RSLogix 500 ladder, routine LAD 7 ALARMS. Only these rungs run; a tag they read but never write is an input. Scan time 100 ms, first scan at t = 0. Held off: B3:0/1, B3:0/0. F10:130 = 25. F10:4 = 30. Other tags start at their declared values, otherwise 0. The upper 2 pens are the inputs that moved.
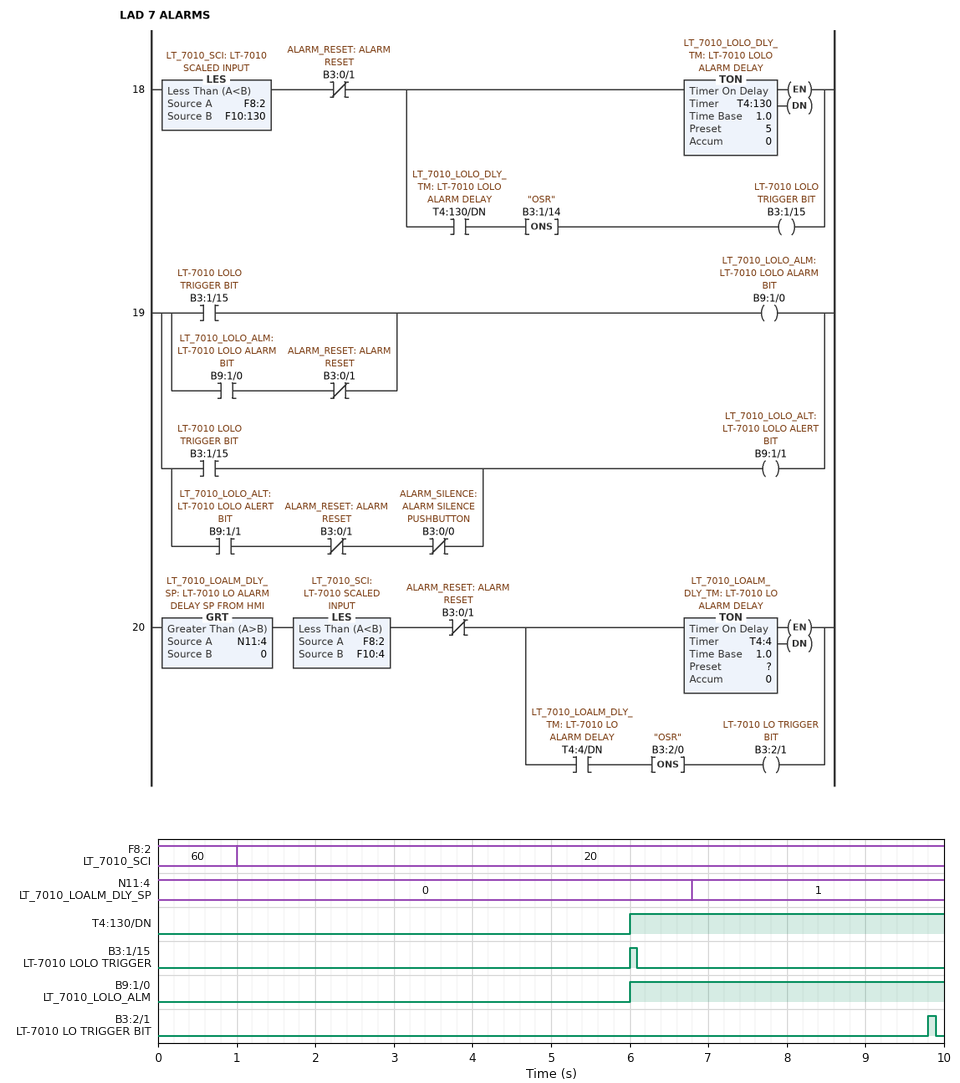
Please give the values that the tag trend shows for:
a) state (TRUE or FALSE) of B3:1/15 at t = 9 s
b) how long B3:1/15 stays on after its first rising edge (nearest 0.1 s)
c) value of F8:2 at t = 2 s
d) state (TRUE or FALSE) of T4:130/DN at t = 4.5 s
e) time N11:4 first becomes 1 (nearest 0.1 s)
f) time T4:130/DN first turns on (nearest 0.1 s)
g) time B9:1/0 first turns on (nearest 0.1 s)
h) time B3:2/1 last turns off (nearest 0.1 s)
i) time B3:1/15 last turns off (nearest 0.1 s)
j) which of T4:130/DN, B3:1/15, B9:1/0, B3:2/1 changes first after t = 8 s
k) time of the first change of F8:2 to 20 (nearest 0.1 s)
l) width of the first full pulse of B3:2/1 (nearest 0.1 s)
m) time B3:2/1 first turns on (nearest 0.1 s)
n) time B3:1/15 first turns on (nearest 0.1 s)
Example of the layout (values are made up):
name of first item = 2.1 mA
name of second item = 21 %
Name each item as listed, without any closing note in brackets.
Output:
state (TRUE or FALSE) of B3:1/15 at t = 9 s = FALSE
how long B3:1/15 stays on after its first rising edge = 0.1 s
value of F8:2 at t = 2 s = 20
state (TRUE or FALSE) of T4:130/DN at t = 4.5 s = FALSE
time N11:4 first becomes 1 = 6.8 s
time T4:130/DN first turns on = 6.0 s
time B9:1/0 first turns on = 6.0 s
time B3:2/1 last turns off = 9.9 s
time B3:1/15 last turns off = 6.1 s
which of T4:130/DN, B3:1/15, B9:1/0, B3:2/1 changes first after t = 8 s = B3:2/1
time of the first change of F8:2 to 20 = 1.0 s
width of the first full pulse of B3:2/1 = 0.1 s
time B3:2/1 first turns on = 9.8 s
time B3:1/15 first turns on = 6.0 s
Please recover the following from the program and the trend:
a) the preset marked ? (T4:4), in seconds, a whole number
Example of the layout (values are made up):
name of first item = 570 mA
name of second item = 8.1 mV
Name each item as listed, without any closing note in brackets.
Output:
the preset marked ? (T4:4), in seconds, a whole number = 3 s
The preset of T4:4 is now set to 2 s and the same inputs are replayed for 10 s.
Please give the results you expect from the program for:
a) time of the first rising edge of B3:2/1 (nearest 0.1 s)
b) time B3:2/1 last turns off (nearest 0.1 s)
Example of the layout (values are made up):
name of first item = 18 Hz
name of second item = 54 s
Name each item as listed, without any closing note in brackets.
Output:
time of the first rising edge of B3:2/1 = 8.8 s
time B3:2/1 last turns off = 8.9 s
